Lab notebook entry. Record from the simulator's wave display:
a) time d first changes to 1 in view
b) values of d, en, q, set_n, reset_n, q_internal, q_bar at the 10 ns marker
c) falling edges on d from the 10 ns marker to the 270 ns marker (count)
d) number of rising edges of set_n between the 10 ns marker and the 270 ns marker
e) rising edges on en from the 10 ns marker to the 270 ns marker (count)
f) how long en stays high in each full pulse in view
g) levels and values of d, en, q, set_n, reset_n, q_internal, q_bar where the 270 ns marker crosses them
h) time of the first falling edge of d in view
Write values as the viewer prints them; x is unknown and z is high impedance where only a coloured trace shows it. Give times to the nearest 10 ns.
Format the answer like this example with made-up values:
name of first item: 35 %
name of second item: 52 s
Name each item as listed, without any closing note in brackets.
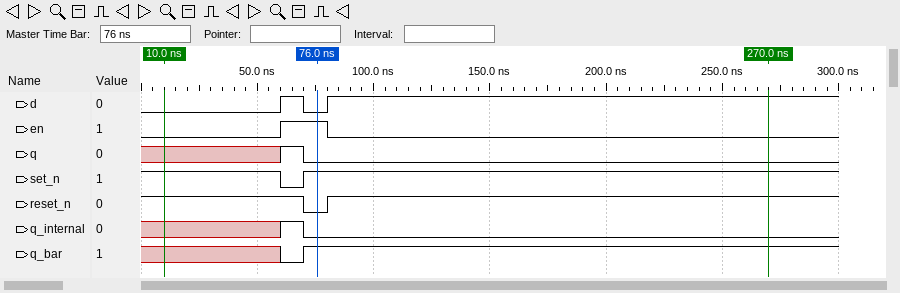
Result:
time d first changes to 1 in view: 60 ns
values of d, en, q, set_n, reset_n, q_internal, q_bar at the 10 ns marker: d=0, en=0, q=x, set_n=1, reset_n=1, q_internal=x, q_bar=x
falling edges on d from the 10 ns marker to the 270 ns marker: 1
number of rising edges of set_n between the 10 ns marker and the 270 ns marker: 1
rising edges on en from the 10 ns marker to the 270 ns marker: 1
how long en stays high in each full pulse in view: 20 ns
levels and values of d, en, q, set_n, reset_n, q_internal, q_bar where the 270 ns marker crosses them: d=1, en=0, q=0, set_n=1, reset_n=1, q_internal=0, q_bar=1
time of the first falling edge of d in view: 70 ns
